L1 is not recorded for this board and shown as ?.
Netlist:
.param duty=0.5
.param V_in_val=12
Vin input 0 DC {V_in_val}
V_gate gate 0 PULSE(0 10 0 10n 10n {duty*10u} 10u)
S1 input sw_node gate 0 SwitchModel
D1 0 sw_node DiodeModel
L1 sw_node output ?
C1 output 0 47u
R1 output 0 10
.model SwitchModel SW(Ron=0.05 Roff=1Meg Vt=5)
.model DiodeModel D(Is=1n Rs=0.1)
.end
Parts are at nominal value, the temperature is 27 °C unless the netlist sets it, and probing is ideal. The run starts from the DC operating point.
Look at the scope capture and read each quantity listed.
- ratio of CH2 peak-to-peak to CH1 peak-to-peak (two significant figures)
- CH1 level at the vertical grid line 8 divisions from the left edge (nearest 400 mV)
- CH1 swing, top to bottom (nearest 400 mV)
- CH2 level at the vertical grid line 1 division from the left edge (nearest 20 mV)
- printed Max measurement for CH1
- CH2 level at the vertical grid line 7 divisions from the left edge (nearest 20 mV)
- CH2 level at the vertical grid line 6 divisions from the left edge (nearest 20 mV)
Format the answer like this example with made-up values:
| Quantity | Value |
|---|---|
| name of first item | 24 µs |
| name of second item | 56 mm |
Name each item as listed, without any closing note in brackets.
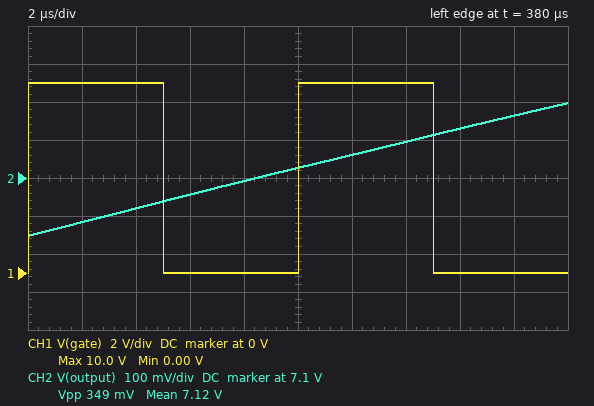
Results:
| Quantity | Value |
|---|---|
| ratio of CH2 peak-to-peak to CH1 peak-to-peak | 0.035 |
| CH1 level at the vertical grid line 8 divisions from the left edge | 0 V |
| CH1 swing, top to bottom | 10.0 V |
| CH2 level at the vertical grid line 1 division from the left edge | 6.98 V |
| printed Max measurement for CH1 | 10.0 V |
| CH2 level at the vertical grid line 7 divisions from the left edge | 7.20 V |
| CH2 level at the vertical grid line 6 divisions from the left edge | 7.16 V |
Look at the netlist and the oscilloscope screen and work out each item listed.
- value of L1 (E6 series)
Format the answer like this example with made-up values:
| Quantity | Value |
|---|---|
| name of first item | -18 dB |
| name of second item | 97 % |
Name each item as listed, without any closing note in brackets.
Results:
| Quantity | Value |
|---|---|
| value of L1 | 680 µH |
